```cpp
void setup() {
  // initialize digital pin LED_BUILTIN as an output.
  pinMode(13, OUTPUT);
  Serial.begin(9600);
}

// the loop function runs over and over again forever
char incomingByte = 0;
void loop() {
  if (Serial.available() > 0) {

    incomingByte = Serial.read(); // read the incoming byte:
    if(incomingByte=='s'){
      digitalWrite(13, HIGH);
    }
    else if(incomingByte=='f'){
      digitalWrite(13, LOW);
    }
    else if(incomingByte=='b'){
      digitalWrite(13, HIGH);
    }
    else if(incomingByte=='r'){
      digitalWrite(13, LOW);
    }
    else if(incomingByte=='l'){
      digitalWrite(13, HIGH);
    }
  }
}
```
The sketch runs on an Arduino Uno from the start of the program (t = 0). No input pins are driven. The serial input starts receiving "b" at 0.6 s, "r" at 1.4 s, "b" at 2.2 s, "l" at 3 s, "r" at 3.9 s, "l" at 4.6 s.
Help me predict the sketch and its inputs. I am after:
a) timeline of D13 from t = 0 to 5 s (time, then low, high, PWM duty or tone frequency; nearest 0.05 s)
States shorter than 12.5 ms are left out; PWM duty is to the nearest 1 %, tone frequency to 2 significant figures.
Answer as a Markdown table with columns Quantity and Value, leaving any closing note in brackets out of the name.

| Quantity | Value |
|---|---|
| timeline of D13 from t = 0 to 5 s | 0 s low; 0.6 s high; 1.4 s low; 2.2 s high; 3.9 s low; 4.6 s high |
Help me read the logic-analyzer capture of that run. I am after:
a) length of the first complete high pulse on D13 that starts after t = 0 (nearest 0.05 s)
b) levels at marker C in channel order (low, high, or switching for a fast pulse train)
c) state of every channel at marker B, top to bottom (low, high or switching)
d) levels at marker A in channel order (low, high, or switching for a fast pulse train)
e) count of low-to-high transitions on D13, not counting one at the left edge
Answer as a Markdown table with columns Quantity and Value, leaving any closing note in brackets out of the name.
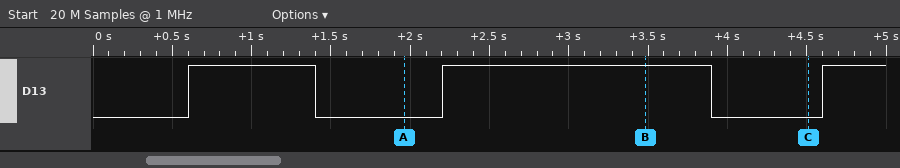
| Quantity | Value |
|---|---|
| length of the first complete high pulse on D13 that starts after t = 0 | 0.80 s |
| levels at marker C in channel order | D13 low |
| state of every channel at marker B, top to bottom | D13 high |
| levels at marker A in channel order | D13 low |
| count of low-to-high transitions on D13, not counting one at the left edge | 3 |
